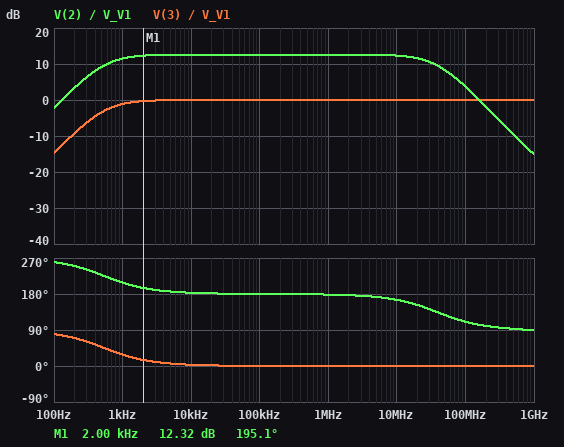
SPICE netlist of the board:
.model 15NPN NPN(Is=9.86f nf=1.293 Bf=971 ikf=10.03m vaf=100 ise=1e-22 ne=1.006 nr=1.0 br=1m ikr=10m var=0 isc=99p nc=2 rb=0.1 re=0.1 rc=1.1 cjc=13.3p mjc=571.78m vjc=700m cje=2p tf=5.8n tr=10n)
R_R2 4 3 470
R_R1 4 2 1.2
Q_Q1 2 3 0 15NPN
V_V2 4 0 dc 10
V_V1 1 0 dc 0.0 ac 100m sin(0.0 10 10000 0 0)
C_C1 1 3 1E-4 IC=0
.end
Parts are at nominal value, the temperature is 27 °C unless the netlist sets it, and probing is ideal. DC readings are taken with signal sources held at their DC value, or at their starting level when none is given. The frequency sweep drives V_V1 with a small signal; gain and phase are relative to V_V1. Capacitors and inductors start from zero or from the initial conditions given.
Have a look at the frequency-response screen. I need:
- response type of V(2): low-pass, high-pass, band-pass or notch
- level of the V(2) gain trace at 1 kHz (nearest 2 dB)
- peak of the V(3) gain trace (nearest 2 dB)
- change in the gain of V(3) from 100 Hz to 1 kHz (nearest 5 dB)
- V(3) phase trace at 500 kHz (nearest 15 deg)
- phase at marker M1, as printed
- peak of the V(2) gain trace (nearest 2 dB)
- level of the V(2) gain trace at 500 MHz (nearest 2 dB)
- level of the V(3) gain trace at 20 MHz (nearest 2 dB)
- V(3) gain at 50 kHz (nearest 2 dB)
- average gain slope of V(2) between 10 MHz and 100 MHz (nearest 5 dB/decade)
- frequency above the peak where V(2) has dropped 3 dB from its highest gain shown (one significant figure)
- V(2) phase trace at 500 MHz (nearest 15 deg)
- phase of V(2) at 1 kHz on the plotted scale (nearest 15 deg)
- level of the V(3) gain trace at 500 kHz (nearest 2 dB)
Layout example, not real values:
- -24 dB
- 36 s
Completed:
- band-pass
- 12 dB
- 0 dB
- 15 dB
- 0 deg
- 195.1 deg
- 12 dB
- -10 dB
- 0 dB
- 0 dB
- -10 dB/decade
- 40 MHz
- 90 deg
- 210 deg
- 0 dB
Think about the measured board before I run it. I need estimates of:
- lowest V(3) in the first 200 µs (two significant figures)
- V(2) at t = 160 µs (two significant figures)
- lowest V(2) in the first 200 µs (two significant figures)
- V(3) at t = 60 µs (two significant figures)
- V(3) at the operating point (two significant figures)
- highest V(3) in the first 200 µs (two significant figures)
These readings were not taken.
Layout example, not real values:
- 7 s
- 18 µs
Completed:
- -17 V
- 10 V
- 5.5 V
- -11 V
- 1.2 V
- 6.6 V
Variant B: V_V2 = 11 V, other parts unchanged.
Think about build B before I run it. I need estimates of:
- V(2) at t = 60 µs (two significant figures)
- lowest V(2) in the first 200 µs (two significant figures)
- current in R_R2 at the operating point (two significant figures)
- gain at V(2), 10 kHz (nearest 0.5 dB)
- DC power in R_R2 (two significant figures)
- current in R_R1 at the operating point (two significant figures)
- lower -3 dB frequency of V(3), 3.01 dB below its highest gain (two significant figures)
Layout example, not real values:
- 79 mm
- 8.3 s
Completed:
- 11 V
- 6.0 V
- 21 mA
- 13.0 dB
- 200 mW
- 440 mA
- 590 Hz
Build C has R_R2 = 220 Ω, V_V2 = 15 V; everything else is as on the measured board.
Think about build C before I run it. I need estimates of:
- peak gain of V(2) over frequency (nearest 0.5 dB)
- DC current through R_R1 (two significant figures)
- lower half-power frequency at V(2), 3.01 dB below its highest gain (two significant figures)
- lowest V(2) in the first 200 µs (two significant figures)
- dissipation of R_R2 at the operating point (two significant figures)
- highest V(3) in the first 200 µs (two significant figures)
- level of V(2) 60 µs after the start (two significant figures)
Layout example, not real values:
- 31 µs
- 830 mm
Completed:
- 14.5 dB
- 760 mA
- 1.3 kHz
- 8.2 V
- 850 mW
- 6.7 V
- 15 V
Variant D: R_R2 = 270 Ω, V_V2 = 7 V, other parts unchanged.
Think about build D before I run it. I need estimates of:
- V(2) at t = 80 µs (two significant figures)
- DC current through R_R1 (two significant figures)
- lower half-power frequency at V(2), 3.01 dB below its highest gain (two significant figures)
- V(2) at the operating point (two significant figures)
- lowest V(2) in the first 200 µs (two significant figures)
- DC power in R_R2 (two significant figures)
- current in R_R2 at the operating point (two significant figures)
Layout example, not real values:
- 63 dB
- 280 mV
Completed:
- 7.0 V
- 430 mA
- 610 Hz
- 6.5 V
- 3.9 V
- 120 mW
- 21 mA
